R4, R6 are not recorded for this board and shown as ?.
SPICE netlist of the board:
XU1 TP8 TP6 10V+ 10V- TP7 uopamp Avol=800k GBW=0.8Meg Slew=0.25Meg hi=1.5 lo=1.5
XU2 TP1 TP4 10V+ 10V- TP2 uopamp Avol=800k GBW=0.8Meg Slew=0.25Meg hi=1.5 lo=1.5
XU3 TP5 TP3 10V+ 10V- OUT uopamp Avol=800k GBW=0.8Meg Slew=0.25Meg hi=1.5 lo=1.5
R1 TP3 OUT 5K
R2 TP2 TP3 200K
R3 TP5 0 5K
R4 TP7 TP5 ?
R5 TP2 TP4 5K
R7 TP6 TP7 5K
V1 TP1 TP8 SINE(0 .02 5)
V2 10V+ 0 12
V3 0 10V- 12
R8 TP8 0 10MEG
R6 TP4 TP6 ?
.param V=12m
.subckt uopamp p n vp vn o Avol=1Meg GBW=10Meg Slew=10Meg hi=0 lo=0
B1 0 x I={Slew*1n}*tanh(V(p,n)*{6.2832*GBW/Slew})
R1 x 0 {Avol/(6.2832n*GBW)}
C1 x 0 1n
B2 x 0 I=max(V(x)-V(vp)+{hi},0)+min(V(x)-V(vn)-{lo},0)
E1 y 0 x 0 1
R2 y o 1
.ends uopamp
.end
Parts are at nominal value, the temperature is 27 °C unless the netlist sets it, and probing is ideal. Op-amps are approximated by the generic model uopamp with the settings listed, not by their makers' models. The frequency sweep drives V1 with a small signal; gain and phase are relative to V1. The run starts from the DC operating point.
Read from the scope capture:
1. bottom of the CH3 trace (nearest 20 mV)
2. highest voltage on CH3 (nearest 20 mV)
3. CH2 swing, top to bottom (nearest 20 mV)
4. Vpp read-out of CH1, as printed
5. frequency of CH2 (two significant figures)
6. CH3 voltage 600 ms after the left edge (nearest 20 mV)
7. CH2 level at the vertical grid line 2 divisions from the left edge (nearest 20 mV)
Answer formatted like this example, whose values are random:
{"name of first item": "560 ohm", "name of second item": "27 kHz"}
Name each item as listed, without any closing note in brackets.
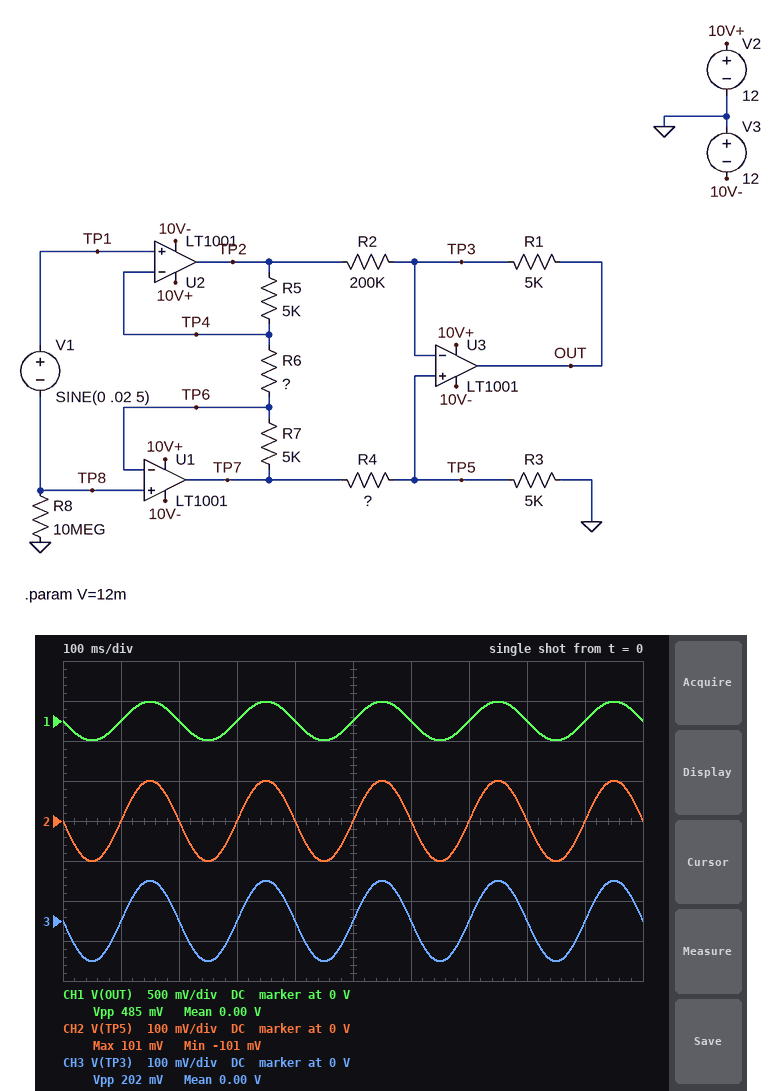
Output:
{"bottom of the CH3 trace": "-100 mV", "highest voltage on CH3": "100 mV", "CH2 swing, top to bottom": "200 mV", "Vpp read-out of CH1, as printed": "485 mV", "frequency of CH2": "5.0 Hz", "CH3 voltage 600 ms after the left edge": "0 V", "CH2 level at the vertical grid line 2 divisions from the left edge": "0 V"}
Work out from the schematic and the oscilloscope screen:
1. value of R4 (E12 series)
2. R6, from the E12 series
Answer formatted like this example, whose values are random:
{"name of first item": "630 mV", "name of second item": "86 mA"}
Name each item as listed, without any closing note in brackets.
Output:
{"value of R4": "270 kΩ", "R6, from the E12 series": "18 Ω"}
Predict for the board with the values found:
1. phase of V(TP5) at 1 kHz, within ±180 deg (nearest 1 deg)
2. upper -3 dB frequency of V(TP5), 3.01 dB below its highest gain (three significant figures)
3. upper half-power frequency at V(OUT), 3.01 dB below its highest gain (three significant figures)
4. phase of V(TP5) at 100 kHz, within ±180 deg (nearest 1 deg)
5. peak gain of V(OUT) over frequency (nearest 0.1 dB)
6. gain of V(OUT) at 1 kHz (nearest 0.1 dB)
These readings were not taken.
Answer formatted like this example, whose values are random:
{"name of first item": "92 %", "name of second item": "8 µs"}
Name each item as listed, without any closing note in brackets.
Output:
{"phase of V(TP5) at 1 kHz, within ±180 deg": "145 deg", "upper -3 dB frequency of V(TP5), 3.01 dB below its highest gain": "1.44 kHz", "upper half-power frequency at V(OUT), 3.01 dB below its highest gain": "1.44 kHz", "phase of V(TP5) at 100 kHz, within ±180 deg": "84 deg", "peak gain of V(OUT) over frequency": "21.7 dB", "gain of V(OUT) at 1 kHz": "20.0 dB"}
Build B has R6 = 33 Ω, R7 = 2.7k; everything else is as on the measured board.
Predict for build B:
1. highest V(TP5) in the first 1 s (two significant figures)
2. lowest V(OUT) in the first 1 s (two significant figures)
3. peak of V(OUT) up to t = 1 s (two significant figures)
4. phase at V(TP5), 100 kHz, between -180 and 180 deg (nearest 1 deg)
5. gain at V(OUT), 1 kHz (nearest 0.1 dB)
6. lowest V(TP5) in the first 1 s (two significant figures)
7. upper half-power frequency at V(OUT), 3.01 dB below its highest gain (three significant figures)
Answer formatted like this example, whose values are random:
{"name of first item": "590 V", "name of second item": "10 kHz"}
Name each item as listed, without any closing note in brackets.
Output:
{"highest V(TP5) in the first 1 s": "30 mV", "lowest V(OUT) in the first 1 s": "-110 mV", "peak of V(OUT) up to t = 1 s": "110 mV", "phase at V(TP5), 100 kHz, between -180 and 180 deg": "85 deg", "gain at V(OUT), 1 kHz": "14.2 dB", "lowest V(TP5) in the first 1 s": "-30 mV", "upper half-power frequency at V(OUT), 3.01 dB below its highest gain": "3.41 kHz"}
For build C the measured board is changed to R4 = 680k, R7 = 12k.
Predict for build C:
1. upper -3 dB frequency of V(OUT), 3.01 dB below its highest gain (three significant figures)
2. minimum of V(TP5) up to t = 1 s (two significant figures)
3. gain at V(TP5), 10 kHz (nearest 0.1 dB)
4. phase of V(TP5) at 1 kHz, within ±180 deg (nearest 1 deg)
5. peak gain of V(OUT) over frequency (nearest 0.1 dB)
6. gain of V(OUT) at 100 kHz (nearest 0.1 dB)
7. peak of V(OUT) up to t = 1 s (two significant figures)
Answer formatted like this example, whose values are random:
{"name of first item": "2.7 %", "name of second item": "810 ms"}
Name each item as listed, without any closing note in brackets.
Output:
{"upper -3 dB frequency of V(OUT), 3.01 dB below its highest gain": "847 Hz", "minimum of V(TP5) up to t = 1 s": "-77 mV", "gain at V(TP5), 10 kHz": "-7.7 dB", "phase of V(TP5) at 1 kHz, within ±180 deg": "130 deg", "peak gain of V(OUT) over frequency": "21.5 dB", "gain of V(OUT) at 100 kHz": "-19.8 dB", "peak of V(OUT) up to t = 1 s": "190 mV"}
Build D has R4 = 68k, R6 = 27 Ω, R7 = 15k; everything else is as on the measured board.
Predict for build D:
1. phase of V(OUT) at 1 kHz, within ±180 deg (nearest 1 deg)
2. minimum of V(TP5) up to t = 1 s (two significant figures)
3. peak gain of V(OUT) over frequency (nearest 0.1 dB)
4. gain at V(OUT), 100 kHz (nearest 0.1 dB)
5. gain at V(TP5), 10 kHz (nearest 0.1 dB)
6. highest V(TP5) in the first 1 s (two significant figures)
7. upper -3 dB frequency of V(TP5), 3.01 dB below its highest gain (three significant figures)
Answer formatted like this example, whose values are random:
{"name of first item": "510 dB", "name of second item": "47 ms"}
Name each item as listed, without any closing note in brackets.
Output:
{"phase of V(OUT) at 1 kHz, within ±180 deg": "137 deg", "minimum of V(TP5) up to t = 1 s": "-720 mV", "peak gain of V(OUT) over frequency": "32.8 dB", "gain at V(OUT), 100 kHz": "-6.7 dB", "gain at V(TP5), 10 kHz": "12.2 dB", "highest V(TP5) in the first 1 s": "720 mV", "upper -3 dB frequency of V(TP5), 3.01 dB below its highest gain": "1.08 kHz"}
